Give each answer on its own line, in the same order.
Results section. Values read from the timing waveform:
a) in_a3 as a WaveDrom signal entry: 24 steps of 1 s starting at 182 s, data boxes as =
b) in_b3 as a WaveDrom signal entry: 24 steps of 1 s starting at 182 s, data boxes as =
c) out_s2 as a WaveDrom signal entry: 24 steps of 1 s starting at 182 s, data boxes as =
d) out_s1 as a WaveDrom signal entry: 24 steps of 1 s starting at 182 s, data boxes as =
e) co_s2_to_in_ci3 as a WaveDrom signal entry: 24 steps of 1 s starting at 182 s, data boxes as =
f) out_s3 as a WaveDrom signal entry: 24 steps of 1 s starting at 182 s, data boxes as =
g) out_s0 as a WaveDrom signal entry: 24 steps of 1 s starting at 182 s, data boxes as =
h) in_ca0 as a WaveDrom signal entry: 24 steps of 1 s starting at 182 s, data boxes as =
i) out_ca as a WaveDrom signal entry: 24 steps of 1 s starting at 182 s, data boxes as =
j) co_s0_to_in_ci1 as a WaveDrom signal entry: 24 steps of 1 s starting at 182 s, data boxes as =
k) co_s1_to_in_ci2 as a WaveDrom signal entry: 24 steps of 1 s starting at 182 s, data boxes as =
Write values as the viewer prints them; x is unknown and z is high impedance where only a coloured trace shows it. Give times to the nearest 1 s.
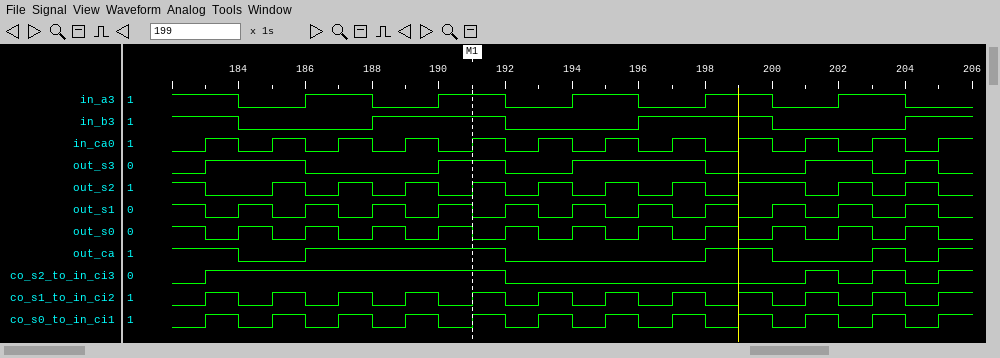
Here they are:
{name: 'in_a3', wave: '1.0.1.0.1.0.1.0.1.0.1.0.'}
{name: 'in_b3', wave: '1.0...1...0...1...0...1.'}
{name: 'out_s2', wave: '10.101010101010101.01010'}
{name: 'out_s1', wave: '101010101010101010101010'}
{name: 'co_s2_to_in_ci3', wave: '01........0........10101'}
{name: 'out_s3', wave: '01..0...1.0.1...0..1.010'}
{name: 'out_s0', wave: '101010101010101010101010'}
{name: 'in_ca0', wave: '010101010101010101010101'}
{name: 'out_ca', wave: '1.0.1.....0.....1.0..101'}
{name: 'co_s0_to_in_ci1', wave: '010101010101010101010101'}
{name: 'co_s1_to_in_ci2', wave: '010101010101010101010101'}
